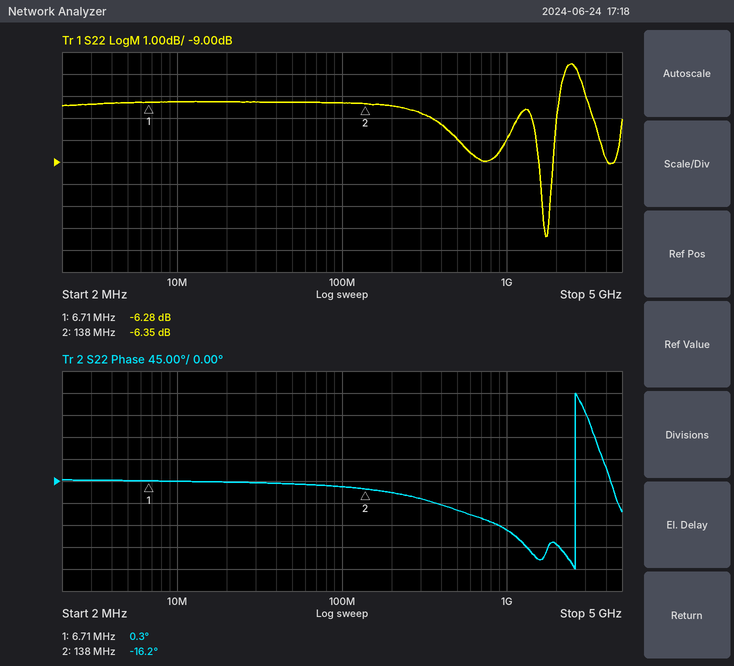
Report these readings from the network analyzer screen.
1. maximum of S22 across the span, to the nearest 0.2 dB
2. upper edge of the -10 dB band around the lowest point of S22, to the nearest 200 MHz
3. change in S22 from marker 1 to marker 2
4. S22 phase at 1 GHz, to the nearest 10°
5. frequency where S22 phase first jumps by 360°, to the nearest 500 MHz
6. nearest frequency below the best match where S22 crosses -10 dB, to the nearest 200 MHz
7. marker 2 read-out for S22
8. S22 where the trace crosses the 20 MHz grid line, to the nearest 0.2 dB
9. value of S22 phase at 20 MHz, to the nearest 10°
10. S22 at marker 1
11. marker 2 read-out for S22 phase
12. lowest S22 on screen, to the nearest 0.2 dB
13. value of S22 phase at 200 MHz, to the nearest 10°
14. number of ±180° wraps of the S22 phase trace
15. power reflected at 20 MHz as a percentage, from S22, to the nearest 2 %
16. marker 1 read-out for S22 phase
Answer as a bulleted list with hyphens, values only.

- -4.6 dB
- 1.8 GHz
- -0.07 dB
- -100°
- 2.5 GHz
- 1.6 GHz
- -6.35 dB
- -6.2 dB
- 0°
- -6.28 dB
- -16.2°
- -12.4 dB
- -20°
- 1
- 24 %
- 0.3°
